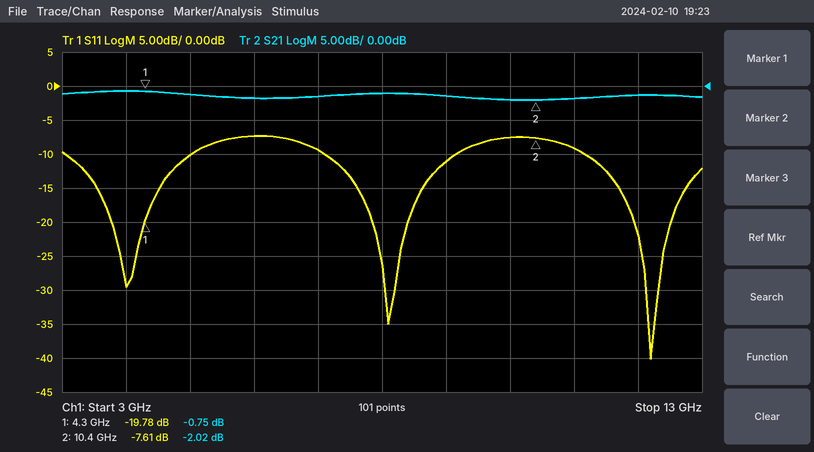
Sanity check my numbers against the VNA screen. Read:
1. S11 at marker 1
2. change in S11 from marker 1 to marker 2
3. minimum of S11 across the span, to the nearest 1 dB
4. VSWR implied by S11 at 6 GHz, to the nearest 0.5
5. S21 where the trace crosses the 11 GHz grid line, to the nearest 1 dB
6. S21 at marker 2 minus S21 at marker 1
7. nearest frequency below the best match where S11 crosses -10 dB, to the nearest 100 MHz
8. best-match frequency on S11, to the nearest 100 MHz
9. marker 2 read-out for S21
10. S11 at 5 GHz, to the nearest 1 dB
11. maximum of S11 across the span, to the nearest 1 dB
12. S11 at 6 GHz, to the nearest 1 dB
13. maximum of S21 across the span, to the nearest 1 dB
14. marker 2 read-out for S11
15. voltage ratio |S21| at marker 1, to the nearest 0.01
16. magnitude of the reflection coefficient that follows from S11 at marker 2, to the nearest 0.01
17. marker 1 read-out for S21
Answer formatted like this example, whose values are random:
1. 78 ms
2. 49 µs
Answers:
1. -19.78 dB
2. 12.17 dB
3. -40 dB
4. 2.5
5. -2 dB
6. -1.27 dB
7. 11.2 GHz
8. 12.2 GHz
9. -2.02 dB
10. -10 dB
11. -7 dB
12. -7 dB
13. -1 dB
14. -7.61 dB
15. 0.92
16. 0.42
17. -0.75 dB
